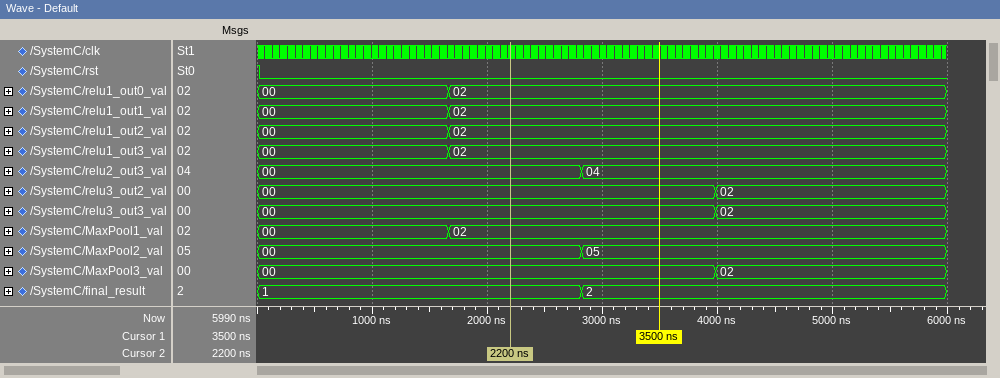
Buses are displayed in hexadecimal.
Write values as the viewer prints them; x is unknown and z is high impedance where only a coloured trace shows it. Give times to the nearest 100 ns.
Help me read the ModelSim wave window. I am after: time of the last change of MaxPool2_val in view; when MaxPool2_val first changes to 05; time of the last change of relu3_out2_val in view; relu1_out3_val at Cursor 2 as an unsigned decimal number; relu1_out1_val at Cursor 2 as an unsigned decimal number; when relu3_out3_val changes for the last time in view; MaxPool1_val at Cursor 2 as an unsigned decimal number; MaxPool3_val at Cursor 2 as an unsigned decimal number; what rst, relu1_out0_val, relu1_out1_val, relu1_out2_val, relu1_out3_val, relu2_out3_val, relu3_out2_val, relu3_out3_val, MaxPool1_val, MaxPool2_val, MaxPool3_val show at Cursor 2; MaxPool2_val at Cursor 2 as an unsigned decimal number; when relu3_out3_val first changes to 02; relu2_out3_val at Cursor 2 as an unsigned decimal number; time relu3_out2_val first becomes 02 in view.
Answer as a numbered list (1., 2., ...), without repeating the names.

1. 2800 ns
2. 2800 ns
3. 4000 ns
4. 2
5. 2
6. 4000 ns
7. 2
8. 0
9. rst=0, relu1_out0_val=02, relu1_out1_val=02, relu1_out2_val=02, relu1_out3_val=02, relu2_out3_val=00, relu3_out2_val=00, relu3_out3_val=00, MaxPool1_val=02, MaxPool2_val=00, MaxPool3_val=00
10. 0
11. 4000 ns
12. 0
13. 4000 ns
